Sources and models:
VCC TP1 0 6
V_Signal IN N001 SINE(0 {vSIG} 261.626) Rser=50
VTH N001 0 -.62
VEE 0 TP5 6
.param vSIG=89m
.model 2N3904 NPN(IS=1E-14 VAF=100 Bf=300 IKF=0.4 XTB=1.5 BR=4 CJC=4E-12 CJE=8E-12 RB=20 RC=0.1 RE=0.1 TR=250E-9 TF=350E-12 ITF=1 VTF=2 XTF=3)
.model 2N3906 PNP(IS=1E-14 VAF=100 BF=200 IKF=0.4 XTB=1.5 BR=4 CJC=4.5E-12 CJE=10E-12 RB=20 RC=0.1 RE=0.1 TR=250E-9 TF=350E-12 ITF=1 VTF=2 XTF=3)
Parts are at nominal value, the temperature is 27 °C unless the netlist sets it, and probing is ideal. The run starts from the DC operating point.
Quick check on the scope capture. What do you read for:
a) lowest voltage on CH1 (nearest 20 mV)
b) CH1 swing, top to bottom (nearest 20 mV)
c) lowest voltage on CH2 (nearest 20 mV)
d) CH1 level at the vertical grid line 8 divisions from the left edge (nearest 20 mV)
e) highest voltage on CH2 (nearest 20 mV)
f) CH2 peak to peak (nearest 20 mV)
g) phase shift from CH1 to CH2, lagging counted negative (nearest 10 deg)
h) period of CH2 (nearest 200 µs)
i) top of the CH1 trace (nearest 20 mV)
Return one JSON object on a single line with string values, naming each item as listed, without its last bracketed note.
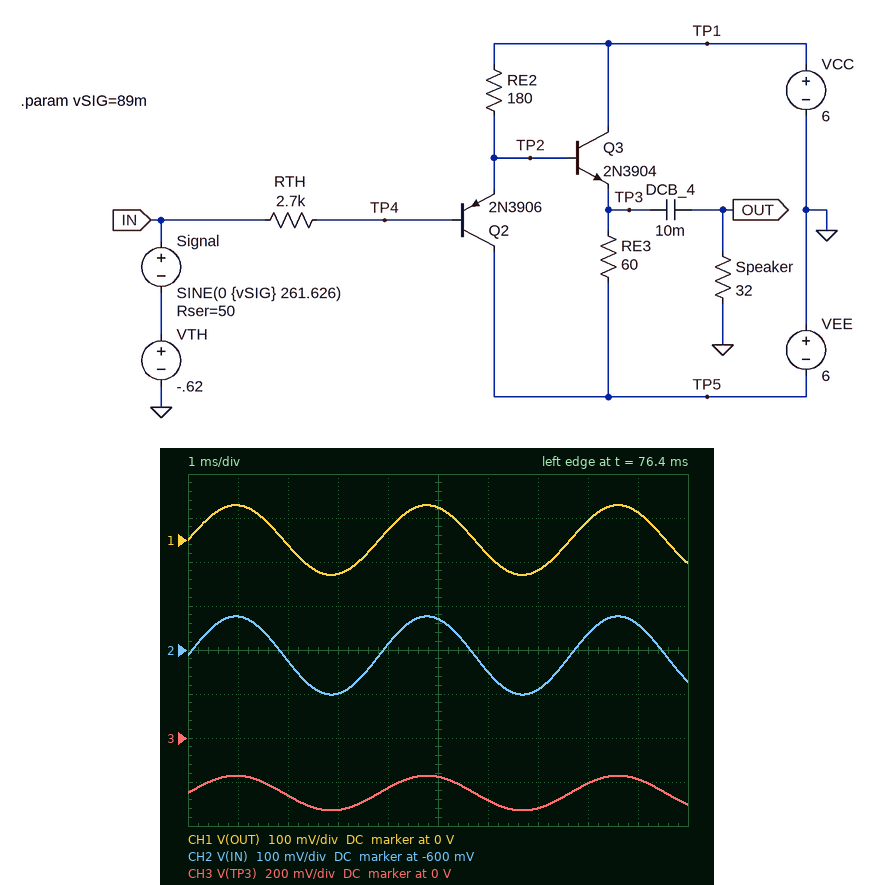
{"lowest voltage on CH1": "-80 mV", "CH1 swing, top to bottom": "160 mV", "lowest voltage on CH2": "-700 mV", "CH1 level at the vertical grid line 8 divisions from the left edge": "40 mV", "highest voltage on CH2": "-520 mV", "CH2 peak to peak": "180 mV", "phase shift from CH1 to CH2, lagging counted negative": "0 deg", "period of CH2": "3.8 ms", "top of the CH1 trace": "80 mV"}
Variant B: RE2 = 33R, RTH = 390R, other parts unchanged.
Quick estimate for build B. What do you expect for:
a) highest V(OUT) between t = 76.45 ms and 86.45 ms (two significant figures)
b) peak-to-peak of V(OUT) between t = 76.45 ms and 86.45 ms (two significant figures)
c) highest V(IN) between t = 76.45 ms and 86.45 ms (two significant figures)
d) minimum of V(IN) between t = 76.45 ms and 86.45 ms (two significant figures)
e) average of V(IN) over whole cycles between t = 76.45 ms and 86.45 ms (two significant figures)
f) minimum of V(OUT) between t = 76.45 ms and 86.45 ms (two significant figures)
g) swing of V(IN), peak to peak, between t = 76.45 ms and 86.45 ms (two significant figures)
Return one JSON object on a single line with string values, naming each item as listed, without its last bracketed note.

{"highest V(OUT) between t = 76.45 ms and 86.45 ms": "77 mV", "peak-to-peak of V(OUT) between t = 76.45 ms and 86.45 ms": "150 mV", "highest V(IN) between t = 76.45 ms and 86.45 ms": "-480 mV", "minimum of V(IN) between t = 76.45 ms and 86.45 ms": "-660 mV", "average of V(IN) over whole cycles between t = 76.45 ms and 86.45 ms": "-570 mV", "minimum of V(OUT) between t = 76.45 ms and 86.45 ms": "-77 mV", "swing of V(IN), peak to peak, between t = 76.45 ms and 86.45 ms": "180 mV"}
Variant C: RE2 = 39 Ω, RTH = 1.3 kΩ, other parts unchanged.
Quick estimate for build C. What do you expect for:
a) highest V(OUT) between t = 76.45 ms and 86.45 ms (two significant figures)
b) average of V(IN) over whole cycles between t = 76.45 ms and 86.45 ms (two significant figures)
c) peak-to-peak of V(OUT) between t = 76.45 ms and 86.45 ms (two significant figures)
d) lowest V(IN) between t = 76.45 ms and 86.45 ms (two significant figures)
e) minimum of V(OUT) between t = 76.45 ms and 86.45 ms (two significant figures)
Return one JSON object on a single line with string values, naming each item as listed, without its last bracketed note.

{"highest V(OUT) between t = 76.45 ms and 86.45 ms": "68 mV", "average of V(IN) over whole cycles between t = 76.45 ms and 86.45 ms": "-580 mV", "peak-to-peak of V(OUT) between t = 76.45 ms and 86.45 ms": "140 mV", "lowest V(IN) between t = 76.45 ms and 86.45 ms": "-670 mV", "minimum of V(OUT) between t = 76.45 ms and 86.45 ms": "-68 mV"}
